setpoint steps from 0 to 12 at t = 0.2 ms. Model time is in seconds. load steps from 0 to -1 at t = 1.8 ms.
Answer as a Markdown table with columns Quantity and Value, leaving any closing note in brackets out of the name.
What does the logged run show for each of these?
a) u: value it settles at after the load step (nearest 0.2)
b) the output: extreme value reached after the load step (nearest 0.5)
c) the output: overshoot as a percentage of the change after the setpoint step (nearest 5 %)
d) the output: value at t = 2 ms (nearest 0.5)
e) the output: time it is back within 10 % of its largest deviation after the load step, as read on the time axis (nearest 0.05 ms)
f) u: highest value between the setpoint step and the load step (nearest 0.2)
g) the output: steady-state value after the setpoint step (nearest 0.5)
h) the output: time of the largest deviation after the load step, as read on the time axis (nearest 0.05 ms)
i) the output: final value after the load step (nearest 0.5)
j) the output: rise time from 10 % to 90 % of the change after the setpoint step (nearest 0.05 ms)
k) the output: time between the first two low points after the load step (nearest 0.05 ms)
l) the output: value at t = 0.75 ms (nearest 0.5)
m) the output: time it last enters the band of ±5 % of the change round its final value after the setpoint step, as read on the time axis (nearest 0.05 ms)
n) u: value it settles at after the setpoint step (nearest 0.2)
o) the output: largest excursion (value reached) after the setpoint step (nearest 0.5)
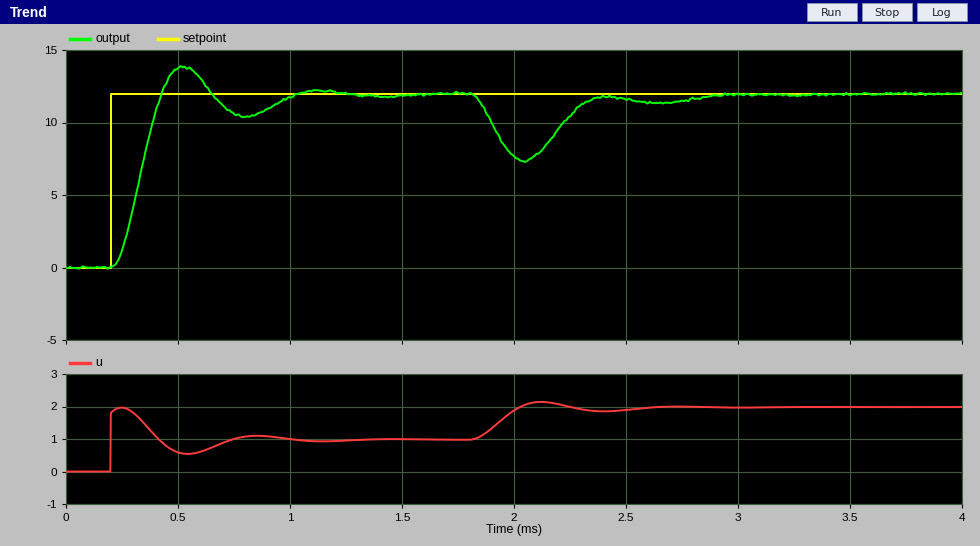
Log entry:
| Quantity | Value |
|---|---|
| u: value it settles at after the load step | 2.0 |
| the output: extreme value reached after the load step | 7.5 |
| the output: overshoot as a percentage of the change after the setpoint step | 15 % |
| the output: value at t = 2 ms | 7.5 |
| the output: time it is back within 10 % of its largest deviation after the load step, as read on the time axis | 2.75 ms |
| u: highest value between the setpoint step and the load step | 2.0 |
| the output: steady-state value after the setpoint step | 12.0 |
| the output: time of the largest deviation after the load step, as read on the time axis | 2.05 ms |
| the output: final value after the load step | 12.0 |
| the output: rise time from 10 % to 90 % of the change after the setpoint step | 0.15 ms |
| the output: time between the first two low points after the load step | 0.60 ms |
| the output: value at t = 0.75 ms | 10.5 |
| the output: time it last enters the band of ±5 % of the change round its final value after the setpoint step, as read on the time axis | 0.95 ms |
| u: value it settles at after the setpoint step | 1.0 |
| the output: largest excursion (value reached) after the setpoint step | 14.0 |
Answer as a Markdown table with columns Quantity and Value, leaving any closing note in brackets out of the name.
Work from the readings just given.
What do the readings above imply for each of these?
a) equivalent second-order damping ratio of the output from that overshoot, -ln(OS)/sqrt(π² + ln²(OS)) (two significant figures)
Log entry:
| Quantity | Value |
|---|---|
| equivalent second-order damping ratio of the output from that overshoot, -ln(OS)/sqrt(π² + ln²(OS)) | 0.52 |
